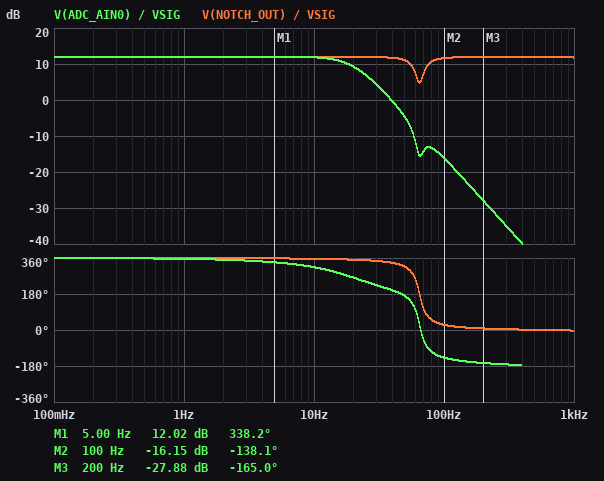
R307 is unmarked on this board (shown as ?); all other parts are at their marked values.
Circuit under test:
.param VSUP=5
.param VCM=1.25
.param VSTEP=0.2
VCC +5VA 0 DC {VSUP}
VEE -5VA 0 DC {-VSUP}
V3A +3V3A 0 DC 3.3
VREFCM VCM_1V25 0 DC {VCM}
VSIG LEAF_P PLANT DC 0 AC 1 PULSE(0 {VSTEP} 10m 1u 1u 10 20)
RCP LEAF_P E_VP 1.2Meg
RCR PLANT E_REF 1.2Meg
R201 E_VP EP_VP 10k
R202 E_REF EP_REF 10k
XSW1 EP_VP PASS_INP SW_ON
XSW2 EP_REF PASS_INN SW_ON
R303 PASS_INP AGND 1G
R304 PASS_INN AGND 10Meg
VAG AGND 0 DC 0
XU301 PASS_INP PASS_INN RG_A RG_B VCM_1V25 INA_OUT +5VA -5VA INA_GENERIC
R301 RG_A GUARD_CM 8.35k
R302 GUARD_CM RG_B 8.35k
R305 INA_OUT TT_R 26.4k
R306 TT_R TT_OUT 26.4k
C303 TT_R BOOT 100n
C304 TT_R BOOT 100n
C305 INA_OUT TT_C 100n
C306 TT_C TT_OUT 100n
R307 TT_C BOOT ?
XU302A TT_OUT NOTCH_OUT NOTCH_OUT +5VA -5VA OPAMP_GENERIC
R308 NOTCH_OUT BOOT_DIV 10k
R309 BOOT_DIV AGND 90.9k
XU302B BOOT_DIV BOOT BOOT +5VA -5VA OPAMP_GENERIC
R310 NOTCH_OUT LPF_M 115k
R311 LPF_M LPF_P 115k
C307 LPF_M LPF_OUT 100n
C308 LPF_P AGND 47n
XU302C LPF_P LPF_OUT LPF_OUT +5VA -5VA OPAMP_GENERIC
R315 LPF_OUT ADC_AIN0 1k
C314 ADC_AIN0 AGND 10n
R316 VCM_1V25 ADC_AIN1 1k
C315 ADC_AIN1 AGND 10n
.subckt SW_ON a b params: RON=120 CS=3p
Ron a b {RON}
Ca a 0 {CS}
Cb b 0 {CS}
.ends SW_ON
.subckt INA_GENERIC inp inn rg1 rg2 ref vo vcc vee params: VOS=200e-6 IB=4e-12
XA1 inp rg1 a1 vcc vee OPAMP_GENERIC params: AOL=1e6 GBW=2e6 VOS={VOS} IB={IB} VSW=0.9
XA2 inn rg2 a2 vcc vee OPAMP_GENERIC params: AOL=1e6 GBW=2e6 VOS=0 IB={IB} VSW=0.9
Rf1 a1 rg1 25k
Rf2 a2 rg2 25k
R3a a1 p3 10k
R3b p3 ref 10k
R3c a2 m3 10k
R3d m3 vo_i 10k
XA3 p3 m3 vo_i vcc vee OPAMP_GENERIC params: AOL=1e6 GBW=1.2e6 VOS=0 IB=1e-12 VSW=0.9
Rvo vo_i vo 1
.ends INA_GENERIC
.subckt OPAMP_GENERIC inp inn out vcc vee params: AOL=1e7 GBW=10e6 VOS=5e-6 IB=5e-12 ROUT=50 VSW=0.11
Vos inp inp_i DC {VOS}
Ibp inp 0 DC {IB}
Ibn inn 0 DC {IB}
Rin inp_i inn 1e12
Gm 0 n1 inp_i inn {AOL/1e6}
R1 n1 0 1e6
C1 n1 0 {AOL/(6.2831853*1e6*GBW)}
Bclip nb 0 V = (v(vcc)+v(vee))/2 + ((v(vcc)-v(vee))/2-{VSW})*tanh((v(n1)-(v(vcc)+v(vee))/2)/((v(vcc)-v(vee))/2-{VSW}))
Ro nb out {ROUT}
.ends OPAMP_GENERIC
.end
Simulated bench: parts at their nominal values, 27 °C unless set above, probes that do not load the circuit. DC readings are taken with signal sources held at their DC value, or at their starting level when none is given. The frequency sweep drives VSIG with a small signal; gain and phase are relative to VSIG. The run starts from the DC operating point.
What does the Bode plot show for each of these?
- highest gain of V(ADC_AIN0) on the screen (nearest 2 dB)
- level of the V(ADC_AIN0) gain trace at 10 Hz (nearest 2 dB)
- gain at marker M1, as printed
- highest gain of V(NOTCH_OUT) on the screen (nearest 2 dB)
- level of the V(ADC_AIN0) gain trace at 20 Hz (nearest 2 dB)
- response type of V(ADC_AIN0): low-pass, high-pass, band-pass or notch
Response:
12 dB
12 dB
12.02 dB
12 dB
10 dB
low-pass
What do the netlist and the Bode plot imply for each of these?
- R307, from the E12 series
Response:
10 kΩ
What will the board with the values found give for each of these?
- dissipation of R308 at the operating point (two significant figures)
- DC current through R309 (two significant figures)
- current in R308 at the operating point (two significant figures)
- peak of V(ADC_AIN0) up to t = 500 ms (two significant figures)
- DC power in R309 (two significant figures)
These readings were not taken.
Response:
1.5 µW
12 µA
12 µA
2.1 V
14 µW
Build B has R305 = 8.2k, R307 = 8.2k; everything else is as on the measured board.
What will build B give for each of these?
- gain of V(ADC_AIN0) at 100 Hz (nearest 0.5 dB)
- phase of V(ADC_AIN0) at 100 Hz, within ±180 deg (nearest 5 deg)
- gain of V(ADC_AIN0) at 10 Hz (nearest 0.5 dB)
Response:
-26.0 dB
-165 deg
12.0 dB
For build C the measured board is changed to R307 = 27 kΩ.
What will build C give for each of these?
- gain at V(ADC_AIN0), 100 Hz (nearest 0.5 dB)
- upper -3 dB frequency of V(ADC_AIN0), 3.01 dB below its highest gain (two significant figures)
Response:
-16.5 dB
20 Hz
